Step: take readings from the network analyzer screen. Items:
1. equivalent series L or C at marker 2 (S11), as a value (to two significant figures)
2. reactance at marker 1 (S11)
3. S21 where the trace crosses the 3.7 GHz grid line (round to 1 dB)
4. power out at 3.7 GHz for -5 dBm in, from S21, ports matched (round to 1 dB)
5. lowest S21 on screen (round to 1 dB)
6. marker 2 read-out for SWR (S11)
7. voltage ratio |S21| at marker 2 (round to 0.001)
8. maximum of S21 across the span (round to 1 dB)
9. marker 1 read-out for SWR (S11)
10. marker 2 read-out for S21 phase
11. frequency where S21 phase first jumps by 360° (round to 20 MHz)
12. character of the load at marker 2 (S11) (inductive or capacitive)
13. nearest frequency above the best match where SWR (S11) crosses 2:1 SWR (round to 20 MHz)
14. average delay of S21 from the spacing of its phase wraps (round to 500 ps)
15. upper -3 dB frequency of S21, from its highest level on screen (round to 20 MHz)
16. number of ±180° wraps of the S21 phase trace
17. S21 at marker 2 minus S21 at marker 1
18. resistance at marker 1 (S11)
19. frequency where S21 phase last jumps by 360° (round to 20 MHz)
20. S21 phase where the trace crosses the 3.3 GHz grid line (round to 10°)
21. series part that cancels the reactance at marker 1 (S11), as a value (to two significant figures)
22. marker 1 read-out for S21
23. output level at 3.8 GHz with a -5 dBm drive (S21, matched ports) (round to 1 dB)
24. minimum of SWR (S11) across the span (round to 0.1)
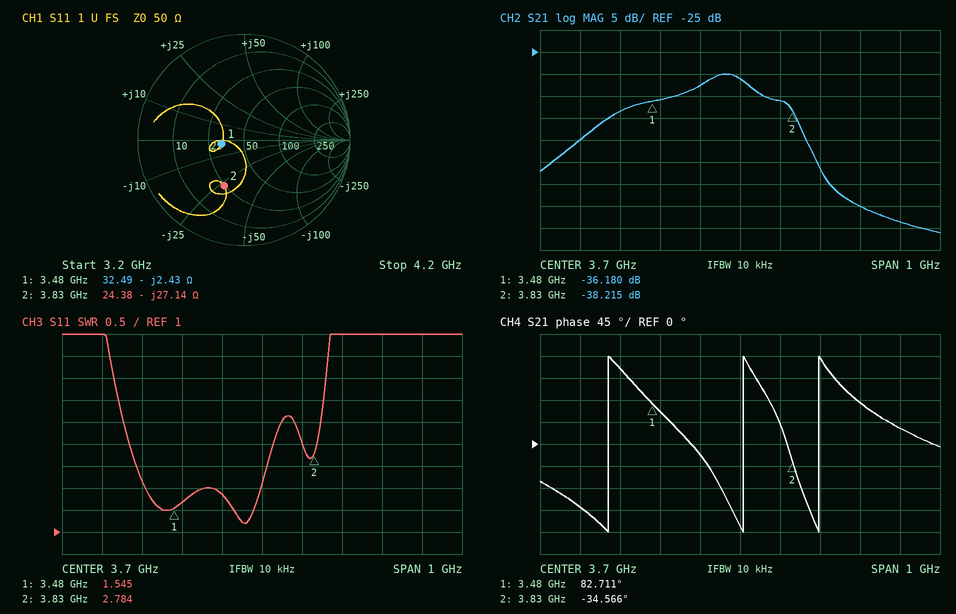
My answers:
1.5 pF
-2.43 Ω
-31 dB
-36 dBm
-66 dB
2.784
0.012
-30 dB
1.545
-34.566°
3.38 GHz
capacitive
3.70 GHz
4.0 ns
3.72 GHz
3
-2.035 dB
32.49 Ω
3.90 GHz
-130°
110 pH
-36.180 dB
-41 dBm
1.2
